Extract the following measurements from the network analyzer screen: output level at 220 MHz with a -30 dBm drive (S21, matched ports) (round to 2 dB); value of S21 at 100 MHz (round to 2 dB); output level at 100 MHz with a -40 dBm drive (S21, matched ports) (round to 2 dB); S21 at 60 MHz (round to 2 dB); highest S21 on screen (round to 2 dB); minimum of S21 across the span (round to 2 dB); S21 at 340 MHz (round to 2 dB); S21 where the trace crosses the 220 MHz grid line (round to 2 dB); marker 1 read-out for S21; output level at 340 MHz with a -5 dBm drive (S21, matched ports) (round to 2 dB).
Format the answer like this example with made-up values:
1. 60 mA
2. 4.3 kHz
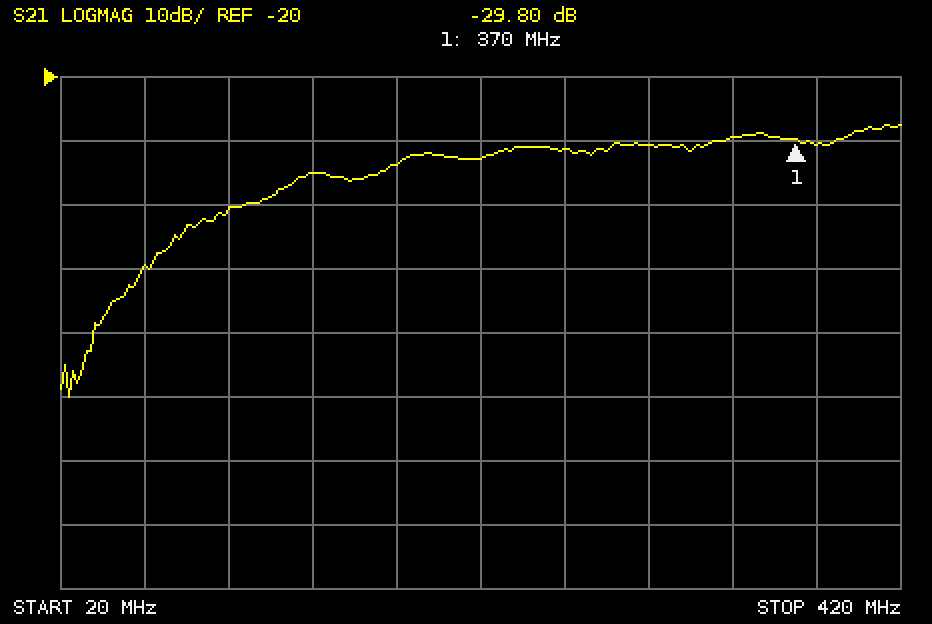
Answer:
1. -62 dBm
2. -40 dB
3. -80 dBm
4. -50 dB
5. -28 dB
6. -70 dB
7. -30 dB
8. -32 dB
9. -29.80 dB
10. -34 dBm
